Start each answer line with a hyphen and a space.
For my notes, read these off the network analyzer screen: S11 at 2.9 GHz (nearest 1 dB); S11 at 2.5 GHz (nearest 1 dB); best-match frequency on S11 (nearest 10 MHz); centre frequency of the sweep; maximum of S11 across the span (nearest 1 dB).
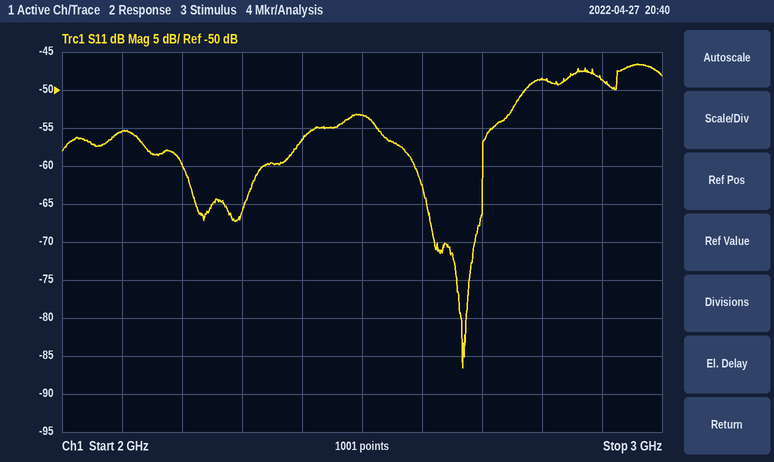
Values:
- -49 dB
- -53 dB
- 2.67 GHz
- 2.5 GHz
- -47 dB
